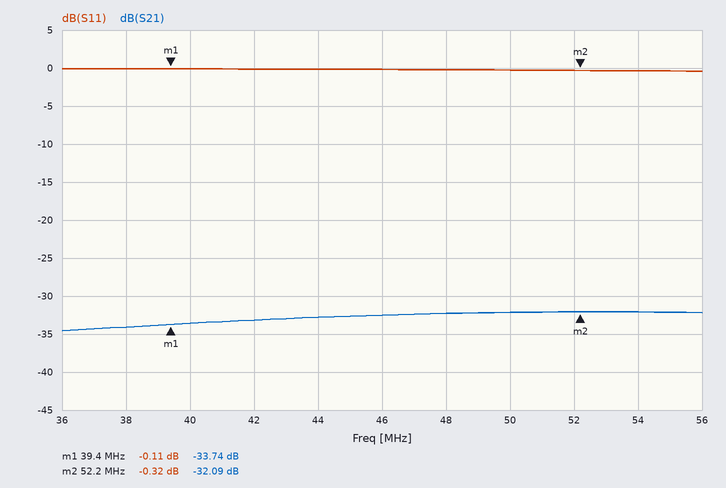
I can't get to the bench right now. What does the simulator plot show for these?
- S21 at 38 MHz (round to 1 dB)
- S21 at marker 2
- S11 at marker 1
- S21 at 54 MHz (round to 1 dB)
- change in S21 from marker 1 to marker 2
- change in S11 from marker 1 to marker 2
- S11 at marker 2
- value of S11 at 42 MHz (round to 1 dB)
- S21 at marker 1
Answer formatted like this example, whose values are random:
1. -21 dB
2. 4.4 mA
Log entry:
1. -34 dB
2. -32.09 dB
3. -0.11 dB
4. -32 dB
5. 1.65 dB
6. -0.21 dB
7. -0.32 dB
8. 0 dB
9. -33.74 dB
